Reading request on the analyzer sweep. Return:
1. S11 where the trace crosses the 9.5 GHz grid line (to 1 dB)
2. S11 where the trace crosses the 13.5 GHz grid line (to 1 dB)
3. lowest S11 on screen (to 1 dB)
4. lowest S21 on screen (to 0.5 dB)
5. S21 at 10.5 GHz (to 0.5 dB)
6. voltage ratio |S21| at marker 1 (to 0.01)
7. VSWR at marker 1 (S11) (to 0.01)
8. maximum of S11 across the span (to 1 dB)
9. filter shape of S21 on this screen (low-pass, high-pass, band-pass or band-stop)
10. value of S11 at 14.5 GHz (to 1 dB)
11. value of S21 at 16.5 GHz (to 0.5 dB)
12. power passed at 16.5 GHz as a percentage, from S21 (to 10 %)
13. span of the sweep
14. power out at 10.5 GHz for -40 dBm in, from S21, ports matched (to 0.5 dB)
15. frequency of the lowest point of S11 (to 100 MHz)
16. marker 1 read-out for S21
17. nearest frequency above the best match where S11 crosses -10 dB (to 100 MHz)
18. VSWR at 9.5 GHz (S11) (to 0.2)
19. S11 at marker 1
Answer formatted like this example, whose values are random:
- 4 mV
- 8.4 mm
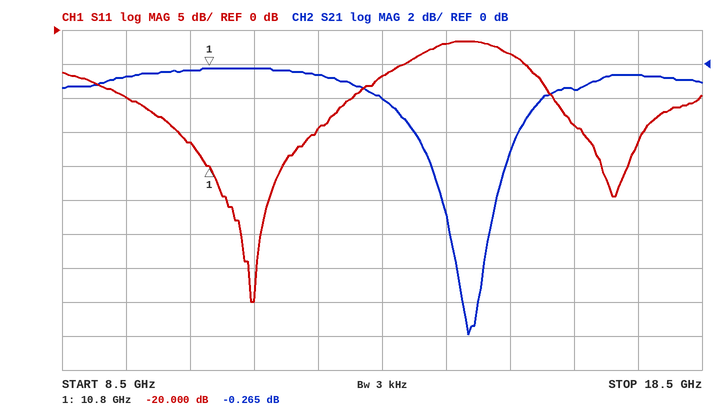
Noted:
- -10 dB
- -7 dB
- -40 dB
- -16.0 dB
- -0.5 dB
- 0.97
- 1.22
- -2 dB
- band-stop
- -2 dB
- -1.5 dB
- 70 %
- 10 GHz
- -40.5 dBm
- 11.5 GHz
- -0.265 dB
- 13.0 GHz
- 2.0
- -20.000 dB
